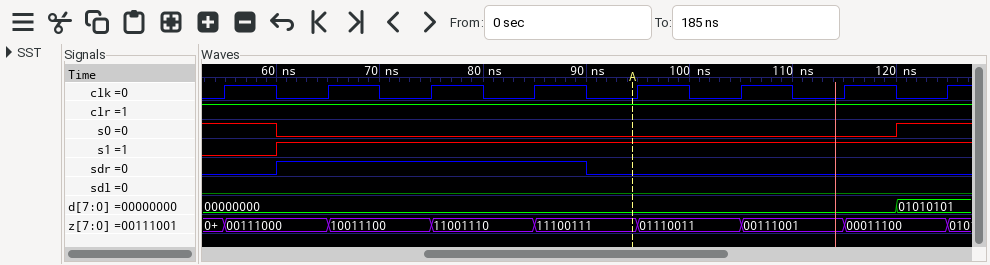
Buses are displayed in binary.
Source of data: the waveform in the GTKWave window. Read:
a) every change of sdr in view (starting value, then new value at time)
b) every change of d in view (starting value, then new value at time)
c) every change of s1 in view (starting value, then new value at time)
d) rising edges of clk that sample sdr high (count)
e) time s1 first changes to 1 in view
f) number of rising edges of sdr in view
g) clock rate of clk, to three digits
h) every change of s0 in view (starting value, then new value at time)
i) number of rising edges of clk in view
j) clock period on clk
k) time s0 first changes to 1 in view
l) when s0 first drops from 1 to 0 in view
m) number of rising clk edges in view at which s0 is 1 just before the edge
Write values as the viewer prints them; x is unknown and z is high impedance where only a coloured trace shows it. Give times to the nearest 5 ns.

0, 1 at 60 ns, 0 at 90 ns
00000000, 01010101 at 120 ns
0, 1 at 60 ns
3
60 ns
1
100 MHz
1, 0 at 60 ns, 1 at 120 ns
8
10 ns
120 ns
60 ns
2
